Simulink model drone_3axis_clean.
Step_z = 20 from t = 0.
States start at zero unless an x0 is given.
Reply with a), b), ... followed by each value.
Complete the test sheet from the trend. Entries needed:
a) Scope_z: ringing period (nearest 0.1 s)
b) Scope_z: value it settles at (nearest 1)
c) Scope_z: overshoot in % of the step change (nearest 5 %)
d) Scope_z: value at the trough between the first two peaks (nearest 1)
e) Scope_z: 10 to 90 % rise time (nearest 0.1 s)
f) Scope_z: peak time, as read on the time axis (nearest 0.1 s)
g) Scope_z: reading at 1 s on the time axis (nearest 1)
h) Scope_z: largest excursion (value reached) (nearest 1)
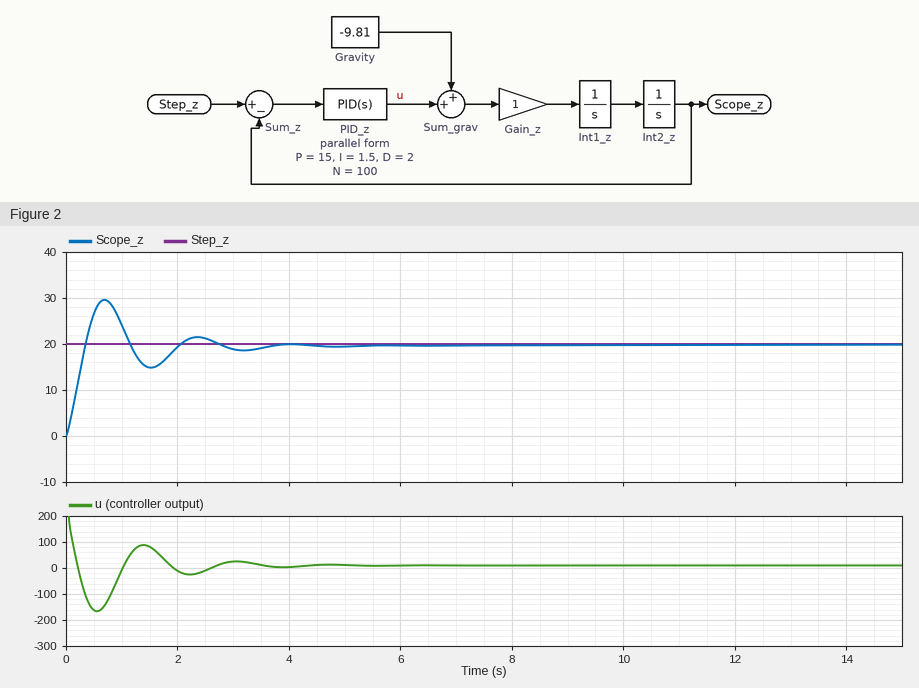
a) 1.7 s
b) 20
c) 50 %
d) 15
e) 0.3 s
f) 0.7 s
g) 24
h) 30
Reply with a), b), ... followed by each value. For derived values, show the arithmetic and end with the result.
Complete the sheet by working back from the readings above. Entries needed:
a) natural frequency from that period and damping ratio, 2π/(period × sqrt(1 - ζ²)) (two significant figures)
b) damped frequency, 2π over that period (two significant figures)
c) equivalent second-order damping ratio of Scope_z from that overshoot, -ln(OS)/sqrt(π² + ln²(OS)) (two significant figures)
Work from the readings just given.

a) 2π / (1.7 × sqrt(1 - 0.22²)) = 3.8 rad/s
b) 2π / 1.7 = 3.7 rad/s
c) ln(0.5) = -0.693; 0.693 / sqrt(9.870 + 0.480) = 0.22
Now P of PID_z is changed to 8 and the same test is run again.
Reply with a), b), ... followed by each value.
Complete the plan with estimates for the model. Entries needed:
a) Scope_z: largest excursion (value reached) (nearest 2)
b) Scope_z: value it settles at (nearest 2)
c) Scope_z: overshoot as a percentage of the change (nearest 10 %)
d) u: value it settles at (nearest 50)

a) 28
b) 20
c) 40 %
d) 0
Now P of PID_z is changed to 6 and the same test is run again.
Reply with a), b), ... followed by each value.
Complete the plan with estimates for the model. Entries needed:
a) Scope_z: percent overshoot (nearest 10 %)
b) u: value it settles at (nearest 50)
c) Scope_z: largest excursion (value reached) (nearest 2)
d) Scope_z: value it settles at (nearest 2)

a) 30 %
b) 0
c) 26
d) 20
